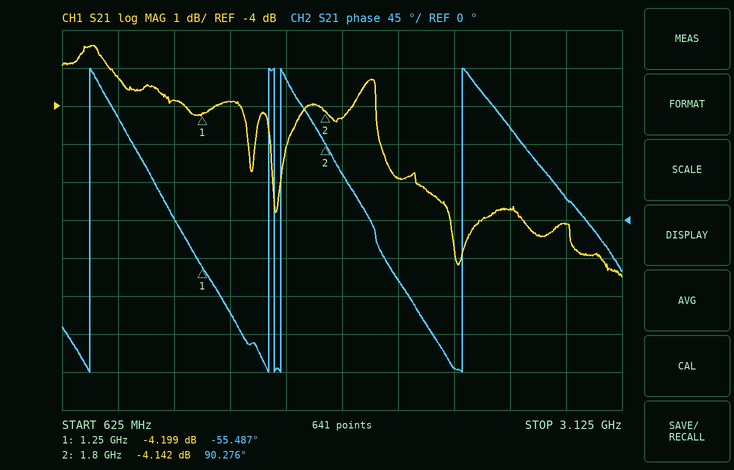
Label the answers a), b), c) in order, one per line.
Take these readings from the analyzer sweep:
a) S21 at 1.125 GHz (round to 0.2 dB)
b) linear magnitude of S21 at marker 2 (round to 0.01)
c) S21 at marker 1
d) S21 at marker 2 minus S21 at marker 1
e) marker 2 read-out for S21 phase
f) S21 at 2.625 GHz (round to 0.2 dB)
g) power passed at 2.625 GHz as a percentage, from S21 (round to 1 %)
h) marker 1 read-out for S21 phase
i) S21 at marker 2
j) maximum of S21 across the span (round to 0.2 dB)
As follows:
a) -3.8 dB
b) 0.62
c) -4.199 dB
d) 0.057 dB
e) 90.276°
f) -6.8 dB
g) 21 %
h) -55.487°
i) -4.142 dB
j) -2.4 dB
